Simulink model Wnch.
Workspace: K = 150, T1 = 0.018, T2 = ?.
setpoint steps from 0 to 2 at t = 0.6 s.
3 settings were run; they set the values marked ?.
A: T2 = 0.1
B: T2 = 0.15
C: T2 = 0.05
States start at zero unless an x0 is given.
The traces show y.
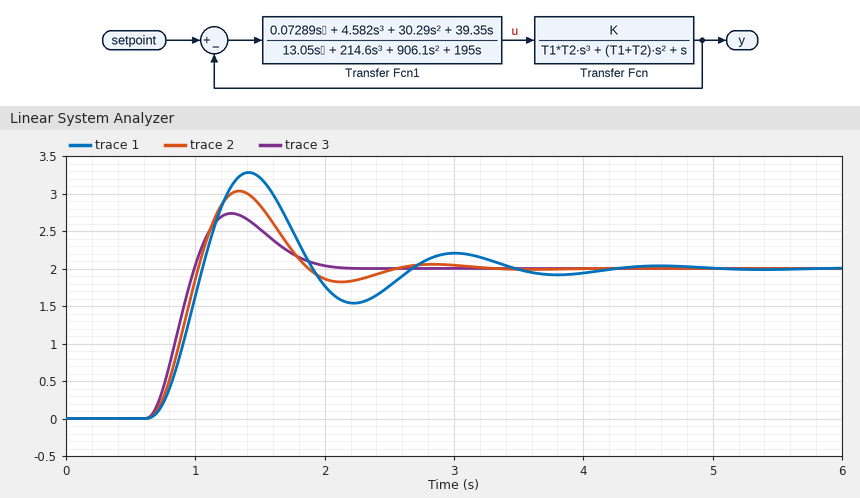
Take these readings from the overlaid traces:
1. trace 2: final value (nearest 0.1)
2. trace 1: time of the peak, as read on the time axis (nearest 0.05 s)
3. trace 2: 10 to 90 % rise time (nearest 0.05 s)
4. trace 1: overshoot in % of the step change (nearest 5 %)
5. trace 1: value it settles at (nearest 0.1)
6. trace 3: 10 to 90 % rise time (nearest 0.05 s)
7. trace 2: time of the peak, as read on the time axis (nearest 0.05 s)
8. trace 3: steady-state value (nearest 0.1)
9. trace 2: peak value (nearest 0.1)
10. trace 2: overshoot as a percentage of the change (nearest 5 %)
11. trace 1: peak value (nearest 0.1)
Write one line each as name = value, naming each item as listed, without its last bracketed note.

trace 2: final value = 2.0
trace 1: time of the peak, as read on the time axis = 1.40 s
trace 2: 10 to 90 % rise time = 0.25 s
trace 1: overshoot in % of the step change = 65 %
trace 1: value it settles at = 2.0
trace 3: 10 to 90 % rise time = 0.25 s
trace 2: time of the peak, as read on the time axis = 1.35 s
trace 3: steady-state value = 2.0
trace 2: peak value = 3.0
trace 2: overshoot as a percentage of the change = 50 %
trace 1: peak value = 3.3
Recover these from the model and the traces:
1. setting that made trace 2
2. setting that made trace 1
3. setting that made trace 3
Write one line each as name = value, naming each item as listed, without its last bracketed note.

setting that made trace 2 = A
setting that made trace 1 = B
setting that made trace 3 = C
